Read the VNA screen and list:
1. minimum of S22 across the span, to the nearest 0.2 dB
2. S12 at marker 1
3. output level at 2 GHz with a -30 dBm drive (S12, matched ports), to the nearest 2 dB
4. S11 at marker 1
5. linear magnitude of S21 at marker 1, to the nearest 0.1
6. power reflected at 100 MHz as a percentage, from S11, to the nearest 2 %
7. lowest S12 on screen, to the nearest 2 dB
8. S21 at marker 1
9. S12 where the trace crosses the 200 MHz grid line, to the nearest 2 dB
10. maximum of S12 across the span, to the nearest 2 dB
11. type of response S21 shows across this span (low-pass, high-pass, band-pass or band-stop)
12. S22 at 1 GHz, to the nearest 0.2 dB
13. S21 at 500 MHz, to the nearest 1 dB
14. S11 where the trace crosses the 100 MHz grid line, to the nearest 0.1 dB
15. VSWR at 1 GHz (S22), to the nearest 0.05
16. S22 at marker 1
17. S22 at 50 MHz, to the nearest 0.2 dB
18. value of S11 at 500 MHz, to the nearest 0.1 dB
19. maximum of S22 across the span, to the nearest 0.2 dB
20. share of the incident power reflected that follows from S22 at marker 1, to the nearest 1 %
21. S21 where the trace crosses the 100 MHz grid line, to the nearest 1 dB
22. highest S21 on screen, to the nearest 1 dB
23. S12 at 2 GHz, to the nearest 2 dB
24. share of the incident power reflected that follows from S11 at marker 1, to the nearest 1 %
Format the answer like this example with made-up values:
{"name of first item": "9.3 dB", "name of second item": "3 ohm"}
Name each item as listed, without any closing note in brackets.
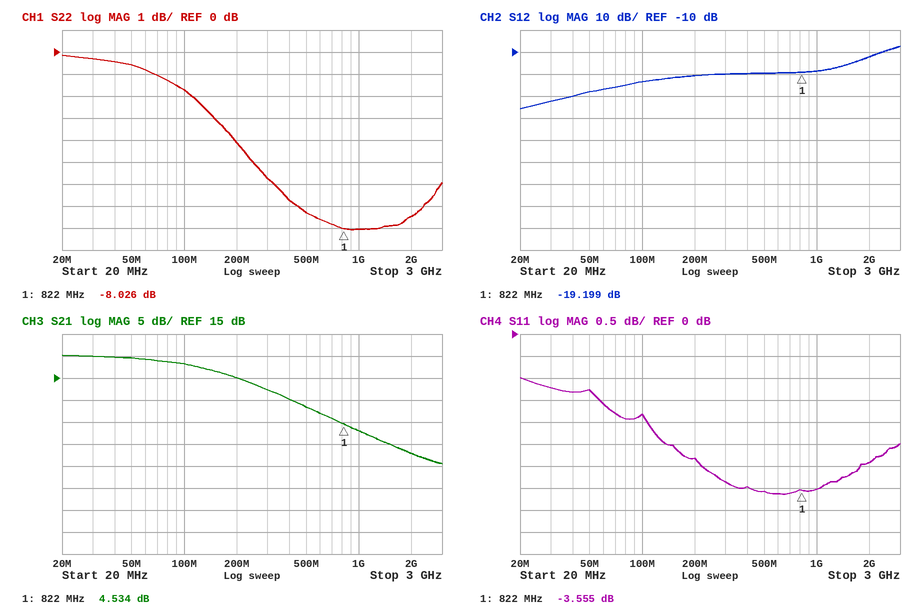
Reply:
{"minimum of S22 across the span, to the nearest 0.2 dB": "-8.0 dB", "S12 at marker 1": "-19.199 dB", "output level at 2 GHz with a -30 dBm drive (S12, matched ports), to the nearest 2 dB": "-42 dBm", "S11 at marker 1": "-3.555 dB", "linear magnitude of S21 at marker 1, to the nearest 0.1": "1.7", "power reflected at 100 MHz as a percentage, from S11, to the nearest 2 %": "66 %", "lowest S12 on screen, to the nearest 2 dB": "-36 dB", "S21 at marker 1": "4.534 dB", "S12 where the trace crosses the 200 MHz grid line, to the nearest 2 dB": "-20 dB", "maximum of S12 across the span, to the nearest 2 dB": "-8 dB", "type of response S21 shows across this span": "low-pass", "S22 at 1 GHz, to the nearest 0.2 dB": "-8.0 dB", "S21 at 500 MHz, to the nearest 1 dB": "8 dB", "S11 where the trace crosses the 100 MHz grid line, to the nearest 0.1 dB": "-1.8 dB", "VSWR at 1 GHz (S22), to the nearest 0.05": "2.30", "S22 at marker 1": "-8.026 dB", "S22 at 50 MHz, to the nearest 0.2 dB": "-0.6 dB", "value of S11 at 500 MHz, to the nearest 0.1 dB": "-3.6 dB", "maximum of S22 across the span, to the nearest 0.2 dB": "-0.2 dB", "share of the incident power reflected that follows from S22 at marker 1, to the nearest 1 %": "16 %", "S21 where the trace crosses the 100 MHz grid line, to the nearest 1 dB": "18 dB", "highest S21 on screen, to the nearest 1 dB": "20 dB", "S12 at 2 GHz, to the nearest 2 dB": "-12 dB", "share of the incident power reflected that follows from S11 at marker 1, to the nearest 1 %": "44 %"}
